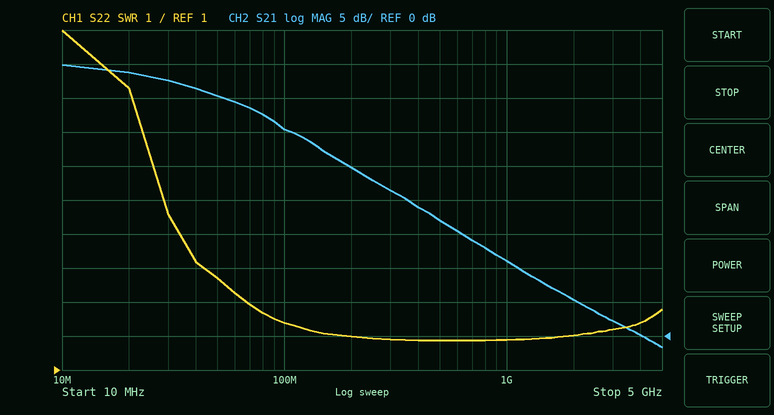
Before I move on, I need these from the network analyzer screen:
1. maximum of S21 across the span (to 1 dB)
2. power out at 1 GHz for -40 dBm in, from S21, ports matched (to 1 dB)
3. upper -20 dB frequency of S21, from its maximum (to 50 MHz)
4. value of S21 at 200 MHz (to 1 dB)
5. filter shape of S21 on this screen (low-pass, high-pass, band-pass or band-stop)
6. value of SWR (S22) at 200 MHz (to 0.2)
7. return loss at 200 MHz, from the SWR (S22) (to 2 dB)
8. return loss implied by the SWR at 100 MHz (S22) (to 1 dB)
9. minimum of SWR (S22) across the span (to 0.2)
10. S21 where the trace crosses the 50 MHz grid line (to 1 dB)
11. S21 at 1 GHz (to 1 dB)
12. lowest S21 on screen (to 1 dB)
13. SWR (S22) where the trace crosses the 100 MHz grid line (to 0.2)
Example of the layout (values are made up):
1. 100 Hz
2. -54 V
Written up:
1. 40 dB
2. -29 dBm
3. 350 MHz
4. 25 dB
5. low-pass
6. 2.0
7. 10 dB
8. 8 dB
9. 1.8
10. 35 dB
11. 11 dB
12. -2 dB
13. 2.4
